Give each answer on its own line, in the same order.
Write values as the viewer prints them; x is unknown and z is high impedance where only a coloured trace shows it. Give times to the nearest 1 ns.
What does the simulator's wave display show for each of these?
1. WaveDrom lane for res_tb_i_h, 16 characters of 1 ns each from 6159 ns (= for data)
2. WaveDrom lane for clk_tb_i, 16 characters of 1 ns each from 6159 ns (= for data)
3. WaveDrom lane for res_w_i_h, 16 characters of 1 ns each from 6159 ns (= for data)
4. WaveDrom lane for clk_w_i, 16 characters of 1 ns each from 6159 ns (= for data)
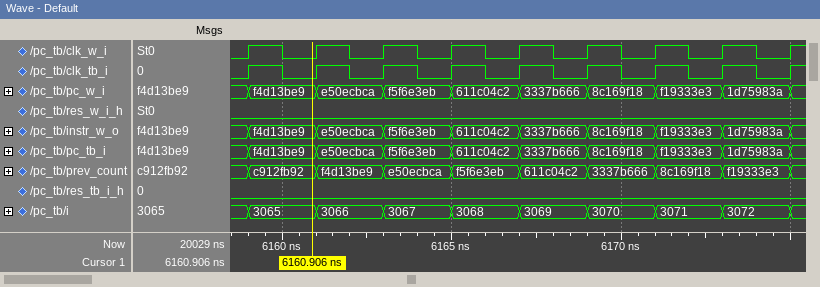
{name: 'res_tb_i_h', wave: '0...............'}
{name: 'clk_tb_i', wave: '1010101010101010'}
{name: 'res_w_i_h', wave: '0...............'}
{name: 'clk_w_i', wave: '1010101010101010'}
